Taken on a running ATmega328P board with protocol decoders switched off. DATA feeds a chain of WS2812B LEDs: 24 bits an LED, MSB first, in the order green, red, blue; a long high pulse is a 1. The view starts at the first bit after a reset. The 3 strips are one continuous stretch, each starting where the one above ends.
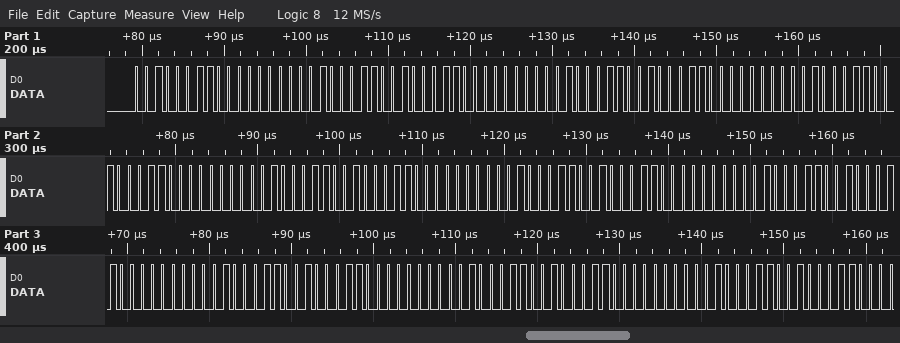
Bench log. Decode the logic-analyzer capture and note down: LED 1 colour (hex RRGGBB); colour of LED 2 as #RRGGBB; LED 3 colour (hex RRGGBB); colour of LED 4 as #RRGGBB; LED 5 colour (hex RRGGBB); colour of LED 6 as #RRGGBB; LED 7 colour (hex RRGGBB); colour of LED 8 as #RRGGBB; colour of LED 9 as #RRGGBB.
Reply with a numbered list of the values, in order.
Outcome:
1. #002323
2. #002323
3. #002323
4. #002323
5. #002323
6. #002323
7. #002323
8. #002323
9. #002323
